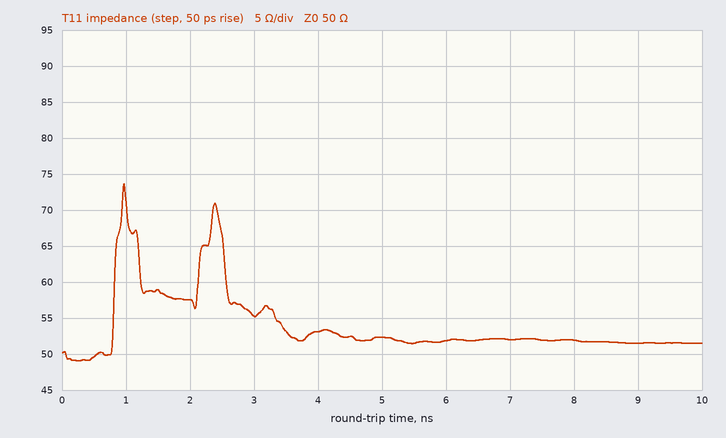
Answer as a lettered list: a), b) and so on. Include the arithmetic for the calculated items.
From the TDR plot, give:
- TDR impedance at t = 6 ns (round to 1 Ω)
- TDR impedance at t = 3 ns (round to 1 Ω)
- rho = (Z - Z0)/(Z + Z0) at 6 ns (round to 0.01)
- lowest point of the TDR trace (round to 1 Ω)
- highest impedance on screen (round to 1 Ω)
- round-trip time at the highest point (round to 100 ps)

a) 52 Ω
b) 55 Ω
c) (52 − 50)/(52 + 50) ≈ +0.02
d) 49 Ω
e) 74 Ω
f) 1.0 ns
